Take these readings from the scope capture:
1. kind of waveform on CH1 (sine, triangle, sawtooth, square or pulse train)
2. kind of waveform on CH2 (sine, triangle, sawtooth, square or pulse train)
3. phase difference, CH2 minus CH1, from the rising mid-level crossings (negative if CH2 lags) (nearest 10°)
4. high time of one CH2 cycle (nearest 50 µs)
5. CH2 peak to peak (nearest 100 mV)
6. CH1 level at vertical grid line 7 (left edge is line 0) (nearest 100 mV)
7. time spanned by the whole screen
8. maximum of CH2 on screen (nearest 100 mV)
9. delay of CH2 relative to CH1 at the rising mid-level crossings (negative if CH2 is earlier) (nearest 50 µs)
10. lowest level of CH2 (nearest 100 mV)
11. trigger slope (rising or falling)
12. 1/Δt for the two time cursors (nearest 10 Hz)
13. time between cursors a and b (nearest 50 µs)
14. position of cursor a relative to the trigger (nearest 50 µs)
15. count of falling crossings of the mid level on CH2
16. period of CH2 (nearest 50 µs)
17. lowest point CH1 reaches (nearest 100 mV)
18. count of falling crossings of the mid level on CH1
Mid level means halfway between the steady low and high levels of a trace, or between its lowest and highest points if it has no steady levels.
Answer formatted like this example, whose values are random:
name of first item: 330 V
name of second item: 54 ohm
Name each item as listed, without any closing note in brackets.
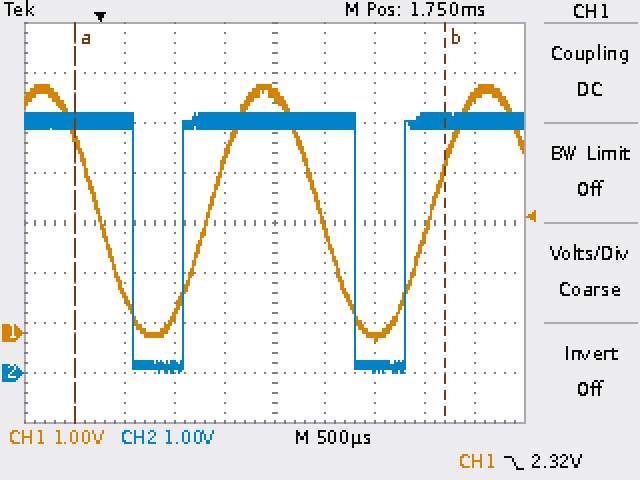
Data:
kind of waveform on CH1: sine
kind of waveform on CH2: pulse train
phase difference, CH2 minus CH1, from the rising mid-level crossings (negative if CH2 lags): +40°
high time of one CH2 cycle: 1.70 ms
CH2 peak to peak: 5.2 V
CH1 level at vertical grid line 7 (left edge is line 0): -100 mV
time spanned by the whole screen: 5 ms
maximum of CH2 on screen: 5.2 V
delay of CH2 relative to CH1 at the rising mid-level crossings (negative if CH2 is earlier): -250 µs
lowest level of CH2: 0.0 V
trigger slope: falling
1/Δt for the two time cursors: 270 Hz
time between cursors a and b: 3.70 ms
position of cursor a relative to the trigger: -250 µs
count of falling crossings of the mid level on CH2: 2
period of CH2: 2.20 ms
lowest point CH1 reaches: -200 mV
count of falling crossings of the mid level on CH1: 2
